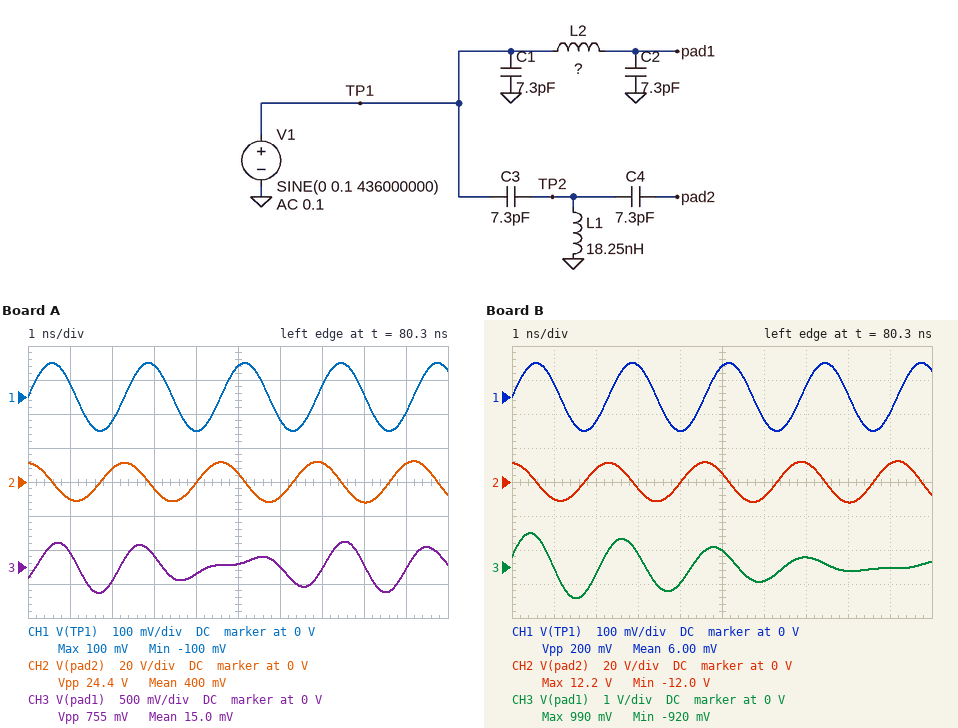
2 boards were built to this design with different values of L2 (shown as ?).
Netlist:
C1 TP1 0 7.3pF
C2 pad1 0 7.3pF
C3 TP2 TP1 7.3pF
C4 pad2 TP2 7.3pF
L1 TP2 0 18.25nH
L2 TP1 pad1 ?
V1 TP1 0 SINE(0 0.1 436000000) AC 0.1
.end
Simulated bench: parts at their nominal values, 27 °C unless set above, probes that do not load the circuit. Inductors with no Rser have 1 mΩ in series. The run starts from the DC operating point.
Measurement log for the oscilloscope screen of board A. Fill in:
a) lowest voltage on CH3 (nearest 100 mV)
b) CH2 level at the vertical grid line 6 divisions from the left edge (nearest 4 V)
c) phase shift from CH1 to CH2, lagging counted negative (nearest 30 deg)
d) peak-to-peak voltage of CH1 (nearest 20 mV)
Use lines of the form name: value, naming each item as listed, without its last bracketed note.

lowest voltage on CH3: -400 mV
CH2 level at the vertical grid line 6 divisions from the left edge: -8 V
phase shift from CH1 to CH2, lagging counted negative: 90 deg
peak-to-peak voltage of CH1: 200 mV
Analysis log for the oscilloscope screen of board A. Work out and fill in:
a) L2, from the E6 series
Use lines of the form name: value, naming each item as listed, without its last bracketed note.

L2, from the E6 series: 10 nH
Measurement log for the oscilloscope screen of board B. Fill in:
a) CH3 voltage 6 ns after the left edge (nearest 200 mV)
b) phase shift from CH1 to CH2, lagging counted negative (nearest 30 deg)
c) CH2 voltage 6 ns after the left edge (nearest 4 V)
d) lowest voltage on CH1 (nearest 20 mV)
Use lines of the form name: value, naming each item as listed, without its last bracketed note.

CH3 voltage 6 ns after the left edge: -400 mV
phase shift from CH1 to CH2, lagging counted negative: 90 deg
CH2 voltage 6 ns after the left edge: -8 V
lowest voltage on CH1: -100 mV
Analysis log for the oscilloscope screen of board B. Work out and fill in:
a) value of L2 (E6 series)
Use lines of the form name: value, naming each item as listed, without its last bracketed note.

value of L2: 15 nH
